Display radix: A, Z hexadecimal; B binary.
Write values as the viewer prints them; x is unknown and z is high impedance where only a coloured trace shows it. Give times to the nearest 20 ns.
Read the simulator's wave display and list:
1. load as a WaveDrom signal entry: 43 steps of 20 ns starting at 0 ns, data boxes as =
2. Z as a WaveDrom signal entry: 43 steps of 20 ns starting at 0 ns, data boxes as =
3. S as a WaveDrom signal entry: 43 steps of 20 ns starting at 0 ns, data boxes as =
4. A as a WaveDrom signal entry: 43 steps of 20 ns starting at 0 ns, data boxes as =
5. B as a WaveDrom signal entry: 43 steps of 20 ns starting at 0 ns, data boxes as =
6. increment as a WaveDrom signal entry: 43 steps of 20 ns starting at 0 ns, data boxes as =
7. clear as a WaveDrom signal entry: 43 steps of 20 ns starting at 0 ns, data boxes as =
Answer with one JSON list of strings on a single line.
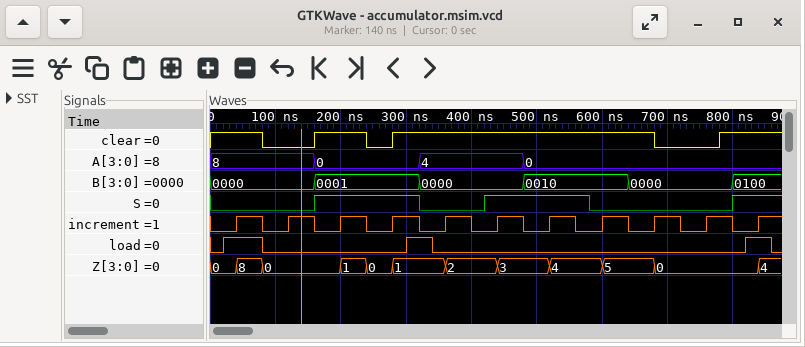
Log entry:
["{name: 'load', wave: '01..0..........1.0.......................1.'}", "{name: 'Z', wave: '=.=.=.....=.=.=...=...=...=...=...=.......=', data: '0 8 0 1 0 1 2 3 4 5 0 4'}", "{name: 'S', wave: '0.......1.......0....1.......0..........1..'}", "{name: 'A', wave: '=.......=.......=.......=..................', data: '8 0 4 0'}", "{name: 'B', wave: '=.......=.......=.......=.......=.......=..', data: '0000 0001 0000 0010 0000 0100'}", "{name: 'increment', wave: '0.1.0.1.0.1.0.1.0.1.0.1.0.1.0.1.0.1.0.1.0.1'}", "{name: 'clear', wave: '1...0...1...0.1...................0....1...'}"]
